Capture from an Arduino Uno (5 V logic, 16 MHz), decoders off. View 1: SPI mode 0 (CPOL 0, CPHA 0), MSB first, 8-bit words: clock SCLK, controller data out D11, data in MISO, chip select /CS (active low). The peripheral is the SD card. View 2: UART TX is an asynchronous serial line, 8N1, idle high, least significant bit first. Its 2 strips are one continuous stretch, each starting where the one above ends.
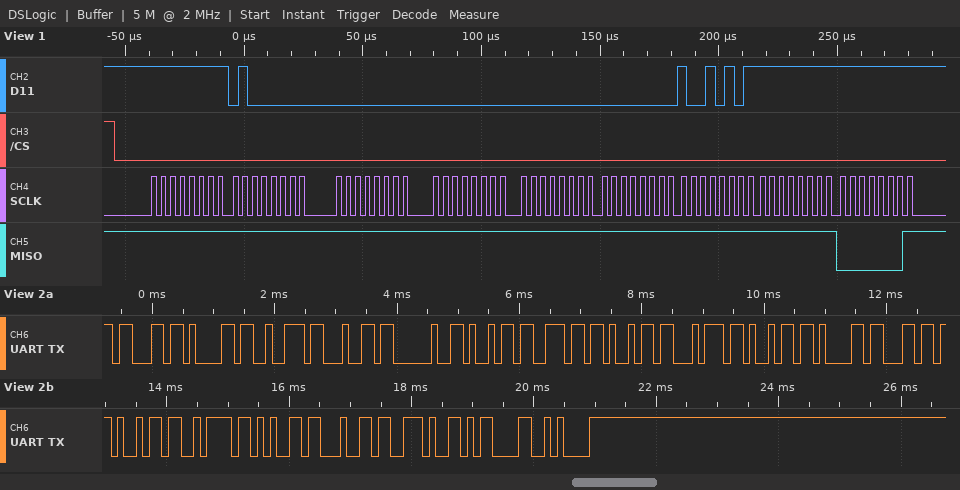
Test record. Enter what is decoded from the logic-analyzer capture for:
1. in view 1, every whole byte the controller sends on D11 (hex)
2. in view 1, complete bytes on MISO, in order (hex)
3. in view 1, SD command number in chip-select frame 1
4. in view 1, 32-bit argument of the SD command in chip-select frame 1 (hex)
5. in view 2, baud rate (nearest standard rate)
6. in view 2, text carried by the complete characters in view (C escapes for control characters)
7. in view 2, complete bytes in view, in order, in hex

0xFF 0x40 0x00 0x00 0x00 0x00 0x95 0xFF 0xFF
0xFF 0xFF 0xFF 0xFF 0xFF 0xFF 0xFF 0xFF 0x01
CMD0
0x00000000
9600 baud
"card initialized.\r\n"
63 61 72 64 20 69 6E 69 74 69 61 6C 69 7A 65 64 2E 0D 0A
